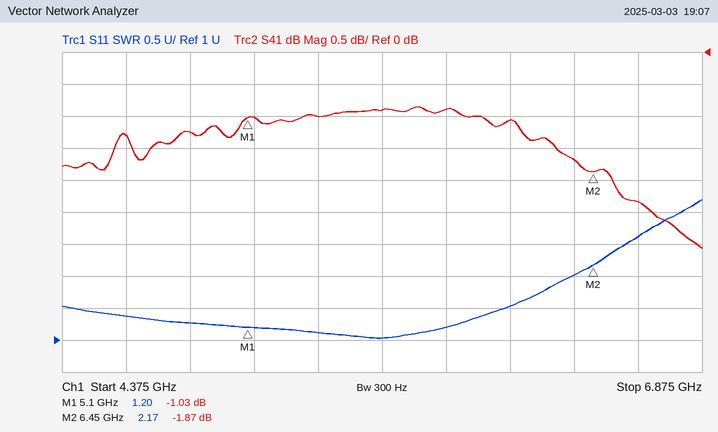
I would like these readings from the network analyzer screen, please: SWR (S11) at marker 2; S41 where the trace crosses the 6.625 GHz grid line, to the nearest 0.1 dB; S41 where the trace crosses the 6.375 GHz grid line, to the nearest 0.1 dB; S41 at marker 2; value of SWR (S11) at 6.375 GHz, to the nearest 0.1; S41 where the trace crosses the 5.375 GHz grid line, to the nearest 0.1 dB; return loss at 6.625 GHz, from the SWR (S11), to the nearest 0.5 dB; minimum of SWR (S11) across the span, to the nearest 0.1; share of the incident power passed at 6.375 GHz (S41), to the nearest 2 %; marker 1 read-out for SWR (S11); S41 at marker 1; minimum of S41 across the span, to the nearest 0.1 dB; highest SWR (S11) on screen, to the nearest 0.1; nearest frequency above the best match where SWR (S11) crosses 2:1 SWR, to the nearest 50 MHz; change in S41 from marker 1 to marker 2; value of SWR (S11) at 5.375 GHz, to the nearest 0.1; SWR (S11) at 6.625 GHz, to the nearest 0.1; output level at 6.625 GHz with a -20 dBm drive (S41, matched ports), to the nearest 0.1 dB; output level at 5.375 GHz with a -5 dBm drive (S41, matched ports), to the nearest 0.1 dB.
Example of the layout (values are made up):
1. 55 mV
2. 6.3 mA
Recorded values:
1. 2.17
2. -2.3 dB
3. -1.7 dB
4. -1.87 dB
5. 2.0
6. -1.0 dB
7. 7.0 dB
8. 1.0
9. 68 %
10. 1.20
11. -1.03 dB
12. -3.1 dB
13. 3.2
14. 6.35 GHz
15. -0.84 dB
16. 1.1
17. 2.6
18. -22.3 dBm
19. -6.0 dBm
